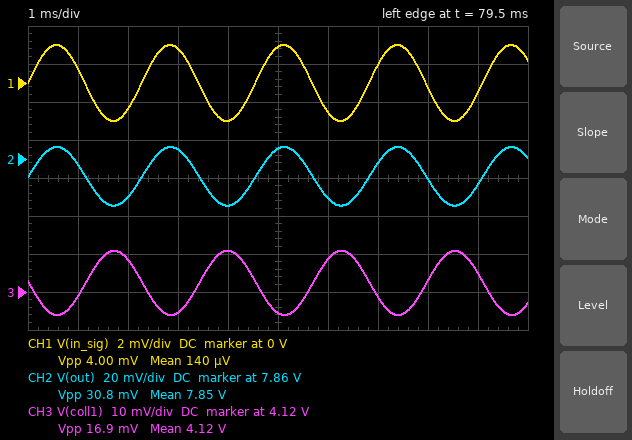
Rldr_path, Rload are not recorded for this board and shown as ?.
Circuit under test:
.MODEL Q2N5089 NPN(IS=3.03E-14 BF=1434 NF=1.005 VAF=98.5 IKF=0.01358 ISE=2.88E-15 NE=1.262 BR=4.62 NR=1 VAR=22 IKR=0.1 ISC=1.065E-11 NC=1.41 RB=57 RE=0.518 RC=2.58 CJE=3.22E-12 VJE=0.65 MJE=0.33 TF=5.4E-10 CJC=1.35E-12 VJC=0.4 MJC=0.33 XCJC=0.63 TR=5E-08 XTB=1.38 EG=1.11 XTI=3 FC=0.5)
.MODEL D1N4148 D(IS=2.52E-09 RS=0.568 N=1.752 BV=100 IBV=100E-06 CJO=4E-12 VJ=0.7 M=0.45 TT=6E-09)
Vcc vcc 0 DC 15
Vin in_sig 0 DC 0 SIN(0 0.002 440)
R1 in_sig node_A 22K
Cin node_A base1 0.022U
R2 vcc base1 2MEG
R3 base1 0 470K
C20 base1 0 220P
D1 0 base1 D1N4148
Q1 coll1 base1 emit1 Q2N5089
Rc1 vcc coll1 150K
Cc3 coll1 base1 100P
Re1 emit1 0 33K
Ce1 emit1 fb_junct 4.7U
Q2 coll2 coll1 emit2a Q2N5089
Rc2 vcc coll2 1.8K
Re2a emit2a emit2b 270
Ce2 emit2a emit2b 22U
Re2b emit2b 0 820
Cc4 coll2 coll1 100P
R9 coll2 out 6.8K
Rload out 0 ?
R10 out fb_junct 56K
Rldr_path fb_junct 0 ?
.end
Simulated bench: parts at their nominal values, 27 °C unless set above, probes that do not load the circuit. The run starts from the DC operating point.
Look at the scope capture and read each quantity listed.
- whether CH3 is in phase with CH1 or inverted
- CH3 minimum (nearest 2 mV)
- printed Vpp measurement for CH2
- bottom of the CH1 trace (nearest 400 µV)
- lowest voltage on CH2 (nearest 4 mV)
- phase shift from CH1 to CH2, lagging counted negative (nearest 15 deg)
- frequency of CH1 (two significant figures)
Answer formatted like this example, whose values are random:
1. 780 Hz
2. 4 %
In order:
1. inverted
2. 4.114 V
3. 30.8 mV
4. -2.0 mV
5. 7.836 V
6. 0 deg
7. 440 Hz
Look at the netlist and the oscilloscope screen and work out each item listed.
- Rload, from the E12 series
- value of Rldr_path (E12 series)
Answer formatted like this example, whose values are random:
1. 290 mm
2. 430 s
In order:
1. 180 kΩ
2. 6.8 kΩ
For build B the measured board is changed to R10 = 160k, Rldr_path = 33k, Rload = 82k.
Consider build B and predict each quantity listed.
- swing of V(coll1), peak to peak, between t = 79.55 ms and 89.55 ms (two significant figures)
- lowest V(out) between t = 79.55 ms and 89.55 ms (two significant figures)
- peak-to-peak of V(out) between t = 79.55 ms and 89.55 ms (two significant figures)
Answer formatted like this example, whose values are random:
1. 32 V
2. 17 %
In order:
1. 12 mV
2. 8.1 V
3. 22 mV
